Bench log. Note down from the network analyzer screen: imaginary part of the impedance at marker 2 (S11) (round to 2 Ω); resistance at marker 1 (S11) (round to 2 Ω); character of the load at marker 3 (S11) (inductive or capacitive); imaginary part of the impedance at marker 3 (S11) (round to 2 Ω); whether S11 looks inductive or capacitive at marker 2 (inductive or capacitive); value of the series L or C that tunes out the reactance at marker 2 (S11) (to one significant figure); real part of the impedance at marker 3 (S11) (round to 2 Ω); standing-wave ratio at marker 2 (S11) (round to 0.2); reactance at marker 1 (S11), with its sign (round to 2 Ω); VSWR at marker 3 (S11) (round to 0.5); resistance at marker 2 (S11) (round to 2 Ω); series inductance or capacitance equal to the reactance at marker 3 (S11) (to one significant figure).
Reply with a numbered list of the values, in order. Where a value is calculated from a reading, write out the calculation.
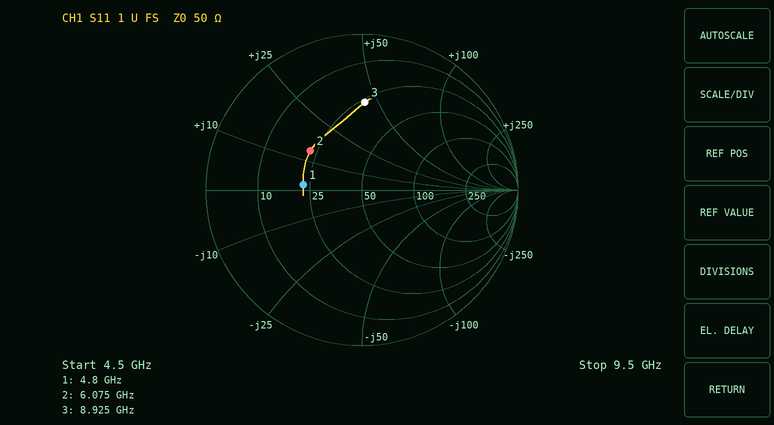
1. +14 Ω
2. 22 Ω
3. inductive
4. +44 Ω
5. inductive
6. C = 1/(2π × 6.075 GHz × 14 Ω) ≈ 2 pF
7. 26 Ω
8. 2.4
9. +2 Ω
10. 3.5
11. 22 Ω
12. L = 44 Ω/(2π × 8.925 GHz) ≈ 785 pH, so 800 pH to one significant figure
